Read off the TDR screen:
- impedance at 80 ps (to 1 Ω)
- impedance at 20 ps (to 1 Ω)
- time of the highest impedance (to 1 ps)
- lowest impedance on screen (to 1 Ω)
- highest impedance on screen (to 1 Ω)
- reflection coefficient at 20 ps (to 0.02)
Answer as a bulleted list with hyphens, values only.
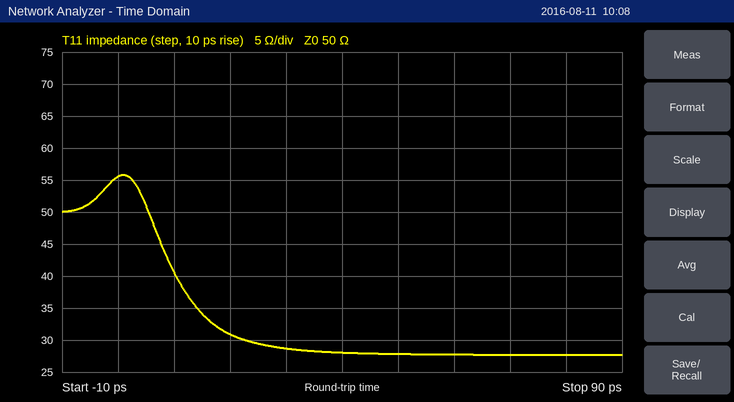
- 28 Ω
- 31 Ω
- 1 ps
- 28 Ω
- 56 Ω
- -0.24
